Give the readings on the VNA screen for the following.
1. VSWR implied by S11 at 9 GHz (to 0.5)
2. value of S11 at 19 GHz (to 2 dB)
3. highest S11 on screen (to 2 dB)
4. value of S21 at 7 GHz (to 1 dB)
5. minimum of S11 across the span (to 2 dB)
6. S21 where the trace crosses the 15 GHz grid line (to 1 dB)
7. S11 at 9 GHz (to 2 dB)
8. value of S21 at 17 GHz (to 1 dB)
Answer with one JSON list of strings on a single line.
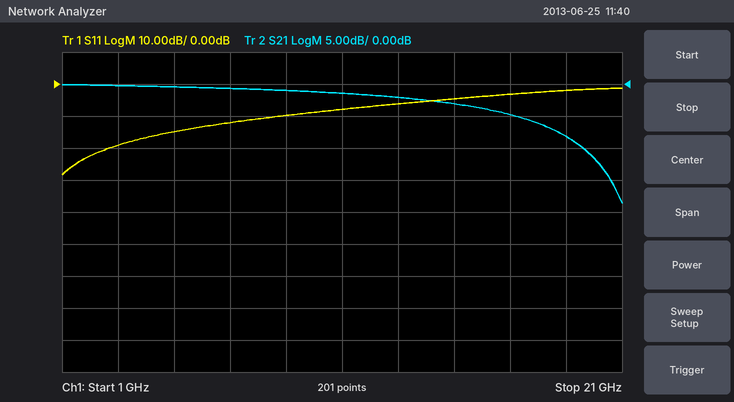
["2.0", "-2 dB", "-2 dB", "-1 dB", "-28 dB", "-3 dB", "-10 dB", "-5 dB"]
